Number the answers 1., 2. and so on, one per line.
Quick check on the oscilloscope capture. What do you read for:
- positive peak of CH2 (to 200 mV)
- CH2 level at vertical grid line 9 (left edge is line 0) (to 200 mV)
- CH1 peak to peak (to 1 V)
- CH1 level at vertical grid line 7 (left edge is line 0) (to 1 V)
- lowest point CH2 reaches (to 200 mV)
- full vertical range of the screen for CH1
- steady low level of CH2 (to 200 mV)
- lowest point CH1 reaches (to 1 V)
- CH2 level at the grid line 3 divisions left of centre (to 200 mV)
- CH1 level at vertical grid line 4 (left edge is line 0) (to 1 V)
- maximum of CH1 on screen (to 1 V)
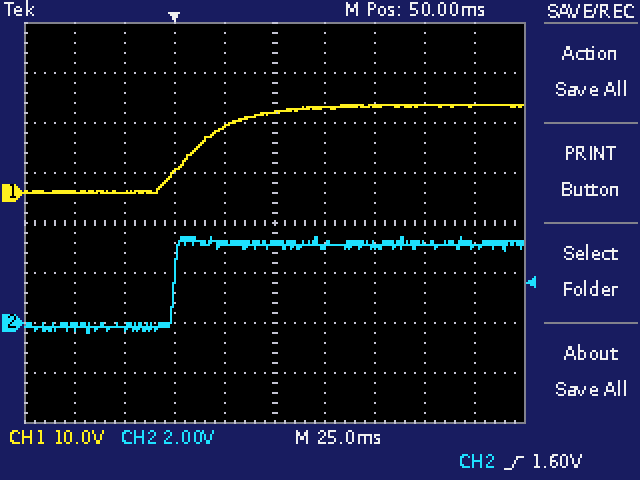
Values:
1. 3.4 V
2. 3.2 V
3. 18 V
4. 17 V
5. -400 mV
6. 80 V
7. -200 mV
8. 0 V
9. -200 mV
10. 13 V
11. 18 V
